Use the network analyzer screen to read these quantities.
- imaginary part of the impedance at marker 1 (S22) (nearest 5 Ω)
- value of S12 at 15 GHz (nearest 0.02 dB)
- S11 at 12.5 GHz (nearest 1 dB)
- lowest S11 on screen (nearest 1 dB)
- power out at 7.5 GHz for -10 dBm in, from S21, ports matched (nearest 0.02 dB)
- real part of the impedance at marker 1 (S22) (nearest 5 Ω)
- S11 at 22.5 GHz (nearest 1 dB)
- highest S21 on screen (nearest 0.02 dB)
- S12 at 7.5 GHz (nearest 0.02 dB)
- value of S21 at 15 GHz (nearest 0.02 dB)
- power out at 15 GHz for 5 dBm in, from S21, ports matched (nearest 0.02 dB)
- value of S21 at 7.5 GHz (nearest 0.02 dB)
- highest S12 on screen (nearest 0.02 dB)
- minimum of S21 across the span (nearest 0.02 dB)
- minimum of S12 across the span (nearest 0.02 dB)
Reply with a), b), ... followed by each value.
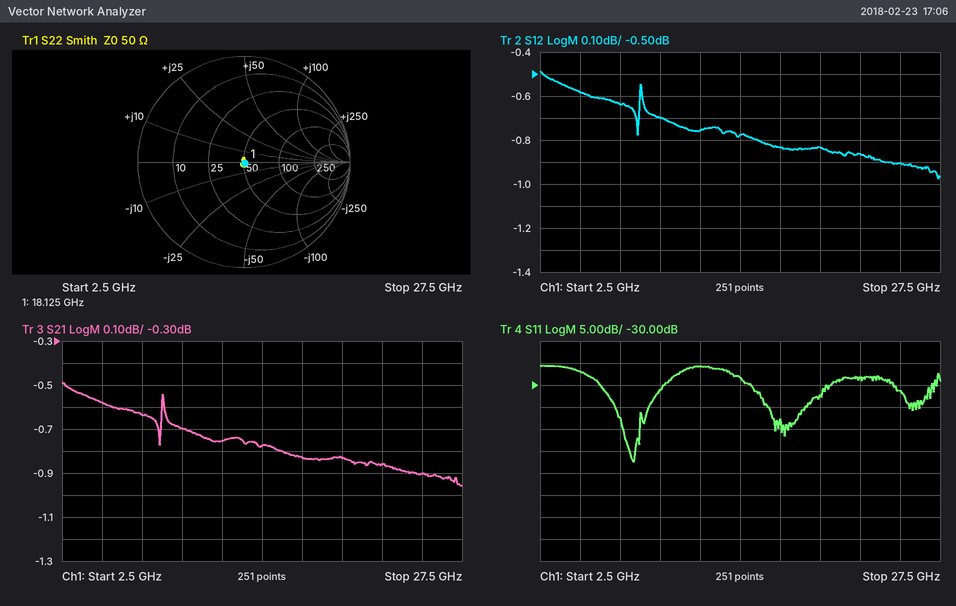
a) 0 Ω
b) -0.78 dB
c) -26 dB
d) -47 dB
e) -10.64 dBm
f) 50 Ω
g) -28 dB
h) -0.48 dB
i) -0.64 dB
j) -0.78 dB
k) 4.22 dBm
l) -0.64 dB
m) -0.48 dB
n) -0.96 dB
o) -0.98 dB
